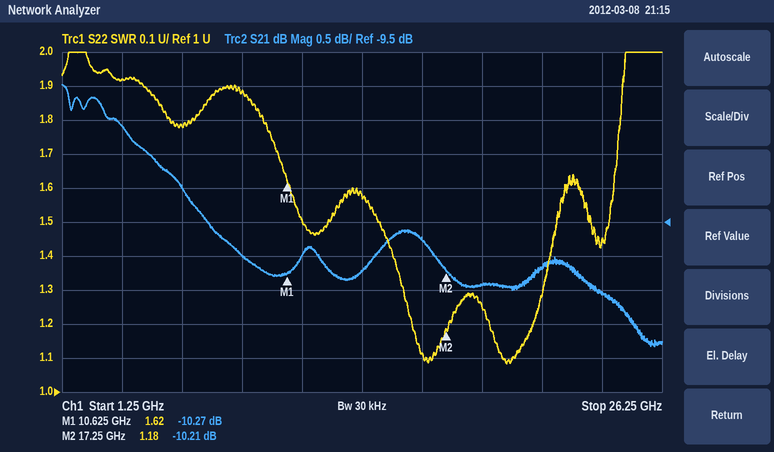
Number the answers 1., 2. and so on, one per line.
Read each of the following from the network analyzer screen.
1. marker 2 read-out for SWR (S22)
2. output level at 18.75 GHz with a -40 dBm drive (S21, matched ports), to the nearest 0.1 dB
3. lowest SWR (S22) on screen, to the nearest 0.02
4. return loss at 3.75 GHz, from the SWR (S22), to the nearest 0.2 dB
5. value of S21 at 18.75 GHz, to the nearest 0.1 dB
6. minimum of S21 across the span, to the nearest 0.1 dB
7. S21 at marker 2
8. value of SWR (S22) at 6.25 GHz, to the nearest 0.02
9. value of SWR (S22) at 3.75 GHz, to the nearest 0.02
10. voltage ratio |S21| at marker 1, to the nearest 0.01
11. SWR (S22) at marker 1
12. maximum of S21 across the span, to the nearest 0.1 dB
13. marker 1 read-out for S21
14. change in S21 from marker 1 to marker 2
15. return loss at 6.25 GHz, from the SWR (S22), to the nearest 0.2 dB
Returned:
1. 1.18
2. -50.4 dBm
3. 1.08
4. 10.0 dB
5. -10.4 dB
6. -11.3 dB
7. -10.21 dB
8. 1.78
9. 1.92
10. 0.31
11. 1.62
12. -7.5 dB
13. -10.27 dB
14. 0.06 dB
15. 11.0 dB
